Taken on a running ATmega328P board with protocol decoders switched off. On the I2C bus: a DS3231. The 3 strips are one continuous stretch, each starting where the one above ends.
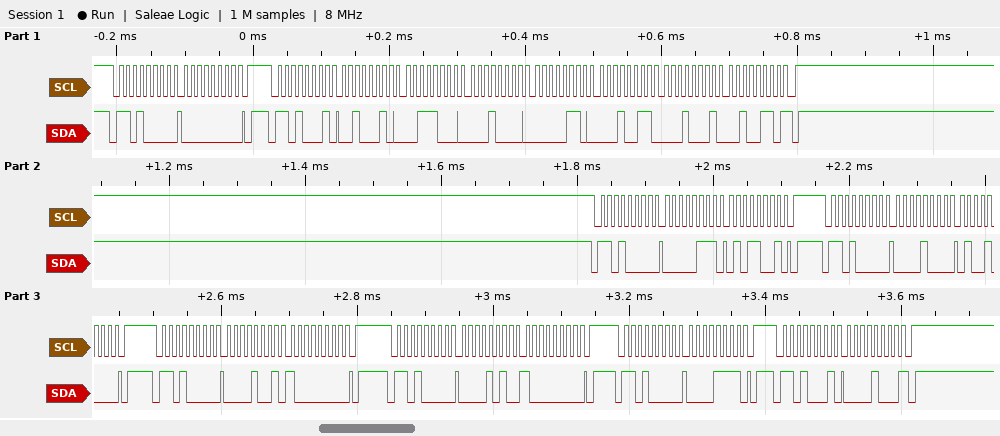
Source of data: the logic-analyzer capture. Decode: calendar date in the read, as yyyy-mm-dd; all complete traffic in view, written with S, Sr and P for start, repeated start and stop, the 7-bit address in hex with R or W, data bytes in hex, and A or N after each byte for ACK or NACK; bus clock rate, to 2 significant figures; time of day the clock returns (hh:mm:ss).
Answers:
2026-11-13
S 68W A 00 A P S 68R A 22 A 38 A 10 A 06 A 13 A 11 A 26 N P S 68W A 07 A 59 A P S 68W A 08 A 48 A P S 68W A 09 A 80 A P S 68W A 0A A 80 A P S 68W A 0F A P S 68R A 08 N P
100 kHz
10:38:22
